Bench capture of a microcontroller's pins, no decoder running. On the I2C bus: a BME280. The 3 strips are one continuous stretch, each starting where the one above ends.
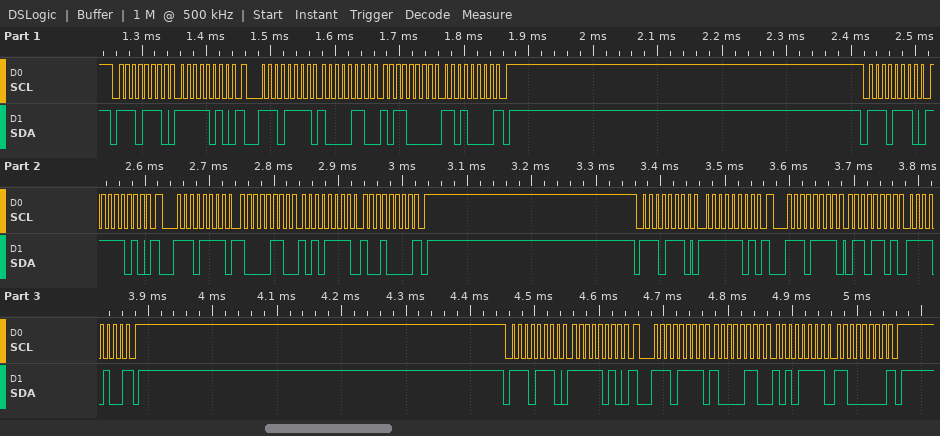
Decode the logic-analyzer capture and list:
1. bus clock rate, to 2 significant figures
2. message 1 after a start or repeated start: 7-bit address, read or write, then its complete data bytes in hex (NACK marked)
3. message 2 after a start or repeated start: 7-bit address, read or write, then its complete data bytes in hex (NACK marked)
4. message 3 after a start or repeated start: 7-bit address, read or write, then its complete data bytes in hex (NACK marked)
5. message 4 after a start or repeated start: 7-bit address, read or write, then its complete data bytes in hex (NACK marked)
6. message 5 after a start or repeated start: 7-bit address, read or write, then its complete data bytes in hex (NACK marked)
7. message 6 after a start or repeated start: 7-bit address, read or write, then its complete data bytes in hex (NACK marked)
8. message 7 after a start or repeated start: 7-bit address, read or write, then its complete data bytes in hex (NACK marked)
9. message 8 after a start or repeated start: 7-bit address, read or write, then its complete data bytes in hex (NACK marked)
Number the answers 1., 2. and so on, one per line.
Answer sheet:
1. 100 kHz
2. 0x77 write: FA
3. 0x77 read: 86 B0 D0 NACK
4. 0x77 write: FA
5. 0x77 read: 86 AF 90 NACK
6. 0x77 write: FD
7. 0x77 read: 6D F4 NACK
8. 0x77 write: FA
9. 0x77 read: 86 AF C0 NACK
